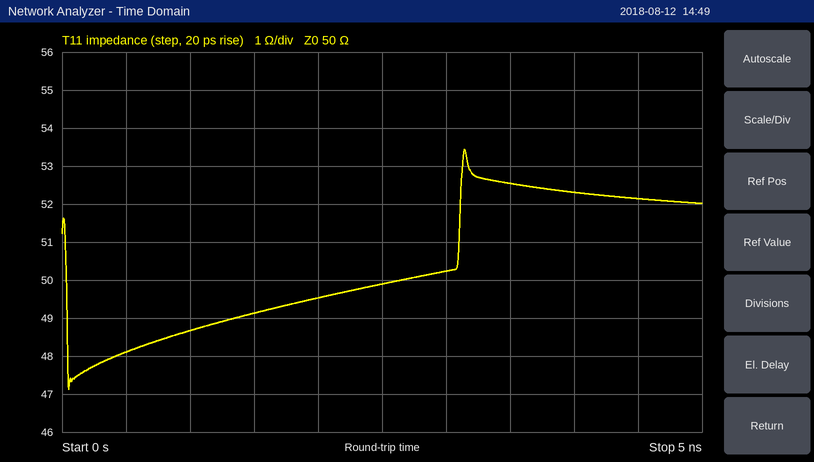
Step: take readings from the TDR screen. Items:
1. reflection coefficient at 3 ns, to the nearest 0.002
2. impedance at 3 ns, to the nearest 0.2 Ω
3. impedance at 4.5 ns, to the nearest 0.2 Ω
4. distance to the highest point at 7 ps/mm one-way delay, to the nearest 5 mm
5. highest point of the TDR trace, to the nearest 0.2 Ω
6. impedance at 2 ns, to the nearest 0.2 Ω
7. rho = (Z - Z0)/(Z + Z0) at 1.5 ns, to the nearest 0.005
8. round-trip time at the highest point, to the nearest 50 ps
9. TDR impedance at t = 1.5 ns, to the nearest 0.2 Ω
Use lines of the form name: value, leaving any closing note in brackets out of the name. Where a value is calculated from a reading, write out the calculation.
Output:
reflection coefficient at 3 ns, to the nearest 0.002: (50.2 − 50)/(50.2 + 50) ≈ +0.002
impedance at 3 ns, to the nearest 0.2 Ω: 50.2 Ω
impedance at 4.5 ns, to the nearest 0.2 Ω: 52.2 Ω
distance to the highest point at 7 ps/mm one-way delay, to the nearest 5 mm: 3.15 ns / 2 / 7 ps/mm ≈ 225 mm
highest point of the TDR trace, to the nearest 0.2 Ω: 53.4 Ω
impedance at 2 ns, to the nearest 0.2 Ω: 49.6 Ω
rho = (Z - Z0)/(Z + Z0) at 1.5 ns, to the nearest 0.005: (49.2 − 50)/(49.2 + 50) ≈ -0.00806, so -0.010 to the nearest 0.005
round-trip time at the highest point, to the nearest 50 ps: 3.15 ns
TDR impedance at t = 1.5 ns, to the nearest 0.2 Ω: 49.2 Ω
